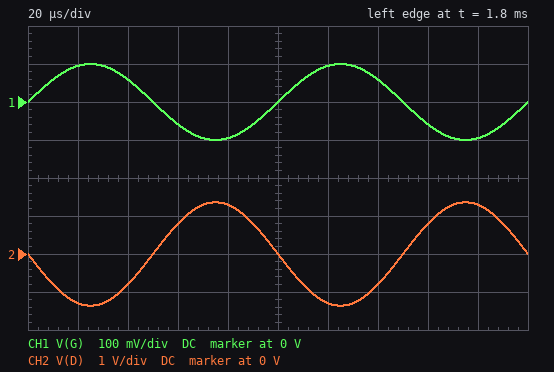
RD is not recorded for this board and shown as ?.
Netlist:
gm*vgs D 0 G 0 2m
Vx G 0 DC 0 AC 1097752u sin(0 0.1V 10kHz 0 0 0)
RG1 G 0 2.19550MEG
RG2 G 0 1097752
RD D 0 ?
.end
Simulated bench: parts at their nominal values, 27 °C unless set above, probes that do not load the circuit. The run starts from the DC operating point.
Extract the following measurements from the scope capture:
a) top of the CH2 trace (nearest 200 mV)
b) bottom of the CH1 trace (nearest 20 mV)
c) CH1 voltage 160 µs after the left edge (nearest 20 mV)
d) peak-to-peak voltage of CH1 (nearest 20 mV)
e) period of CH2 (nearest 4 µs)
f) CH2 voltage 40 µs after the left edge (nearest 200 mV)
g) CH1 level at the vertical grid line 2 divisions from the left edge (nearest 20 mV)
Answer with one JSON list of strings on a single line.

["1.4 V", "-100 mV", "-60 mV", "200 mV", "100 µs", "-800 mV", "60 mV"]
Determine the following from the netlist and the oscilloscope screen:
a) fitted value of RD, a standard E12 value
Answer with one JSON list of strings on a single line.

["6.8 kΩ"]
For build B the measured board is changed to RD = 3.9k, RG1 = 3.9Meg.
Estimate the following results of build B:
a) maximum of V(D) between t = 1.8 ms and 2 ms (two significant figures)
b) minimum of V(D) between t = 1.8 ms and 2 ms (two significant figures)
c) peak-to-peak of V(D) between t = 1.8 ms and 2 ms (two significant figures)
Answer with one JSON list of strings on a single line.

["780 mV", "-780 mV", "1.6 V"]
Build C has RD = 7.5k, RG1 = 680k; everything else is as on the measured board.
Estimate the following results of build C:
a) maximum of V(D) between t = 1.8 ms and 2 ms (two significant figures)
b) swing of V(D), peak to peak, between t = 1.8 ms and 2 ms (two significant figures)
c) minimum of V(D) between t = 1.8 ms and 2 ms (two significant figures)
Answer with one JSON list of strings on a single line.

["1.5 V", "3.0 V", "-1.5 V"]
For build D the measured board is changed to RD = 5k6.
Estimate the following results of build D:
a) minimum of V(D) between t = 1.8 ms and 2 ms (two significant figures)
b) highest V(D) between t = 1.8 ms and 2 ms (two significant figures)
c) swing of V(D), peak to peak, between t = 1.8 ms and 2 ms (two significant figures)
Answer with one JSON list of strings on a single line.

["-1.1 V", "1.1 V", "2.2 V"]
